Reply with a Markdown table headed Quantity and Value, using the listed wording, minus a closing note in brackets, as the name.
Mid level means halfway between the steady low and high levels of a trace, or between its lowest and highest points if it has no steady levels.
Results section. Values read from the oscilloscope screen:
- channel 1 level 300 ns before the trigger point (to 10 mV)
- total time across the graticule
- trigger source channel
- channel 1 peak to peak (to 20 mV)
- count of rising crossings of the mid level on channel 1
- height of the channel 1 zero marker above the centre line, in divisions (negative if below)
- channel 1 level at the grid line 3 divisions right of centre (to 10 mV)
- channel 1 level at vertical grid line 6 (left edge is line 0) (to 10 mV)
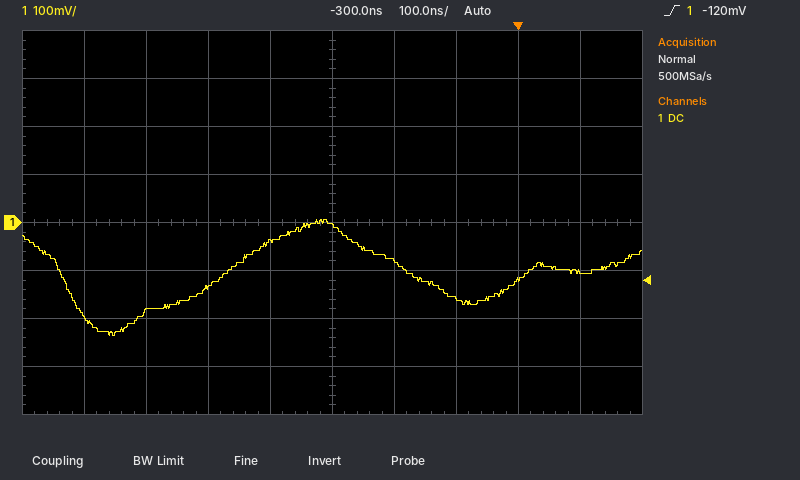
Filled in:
| Quantity | Value |
|---|---|
| channel 1 level 300 ns before the trigger point | -10 mV |
| total time across the graticule | 1 µs |
| trigger source channel | channel 1 |
| channel 1 peak to peak | 240 mV |
| count of rising crossings of the mid level on channel 1 | 2 |
| height of the channel 1 zero marker above the centre line, in divisions | 0.0 div |
| channel 1 level at the grid line 3 divisions right of centre | -120 mV |
| channel 1 level at vertical grid line 6 (left edge is line 0) | -80 mV |
